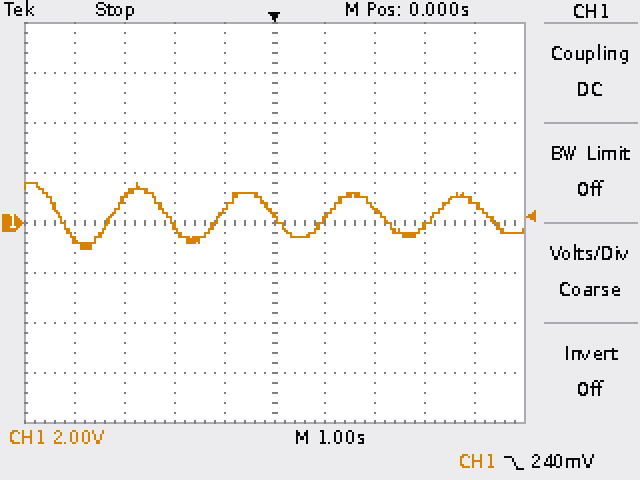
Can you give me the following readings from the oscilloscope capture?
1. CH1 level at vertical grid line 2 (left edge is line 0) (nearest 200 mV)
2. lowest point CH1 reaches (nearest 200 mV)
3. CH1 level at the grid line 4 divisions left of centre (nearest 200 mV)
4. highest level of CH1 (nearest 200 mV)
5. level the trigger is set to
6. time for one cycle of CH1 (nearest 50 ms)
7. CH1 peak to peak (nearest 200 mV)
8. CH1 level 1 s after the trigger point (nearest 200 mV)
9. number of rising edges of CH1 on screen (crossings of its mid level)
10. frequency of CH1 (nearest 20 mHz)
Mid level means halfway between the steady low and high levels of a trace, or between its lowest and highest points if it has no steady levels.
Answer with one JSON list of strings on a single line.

["1.0 V", "-1.0 V", "-600 mV", "1.6 V", "240 mV", "2.15 s", "2.6 V", "200 mV", "4", "460 mHz"]
